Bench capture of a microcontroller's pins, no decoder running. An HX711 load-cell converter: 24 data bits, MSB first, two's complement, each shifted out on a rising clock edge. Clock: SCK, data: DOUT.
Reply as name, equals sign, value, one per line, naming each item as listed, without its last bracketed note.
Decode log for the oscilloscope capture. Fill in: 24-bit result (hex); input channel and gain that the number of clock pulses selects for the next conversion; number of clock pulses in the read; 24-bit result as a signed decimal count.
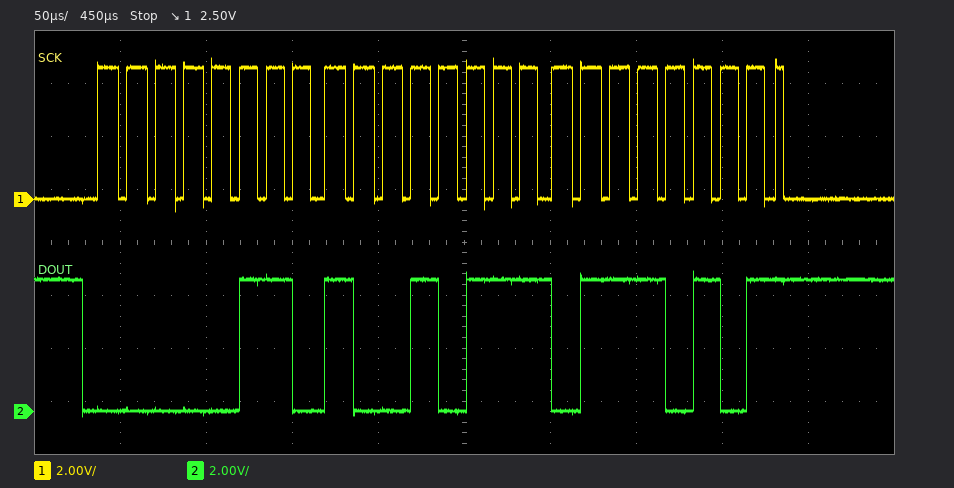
24-bit result = 0x069775
input channel and gain that the number of clock pulses selects for the next conversion = channel A, gain 128
number of clock pulses in the read = 25
24-bit result as a signed decimal count = 431989
